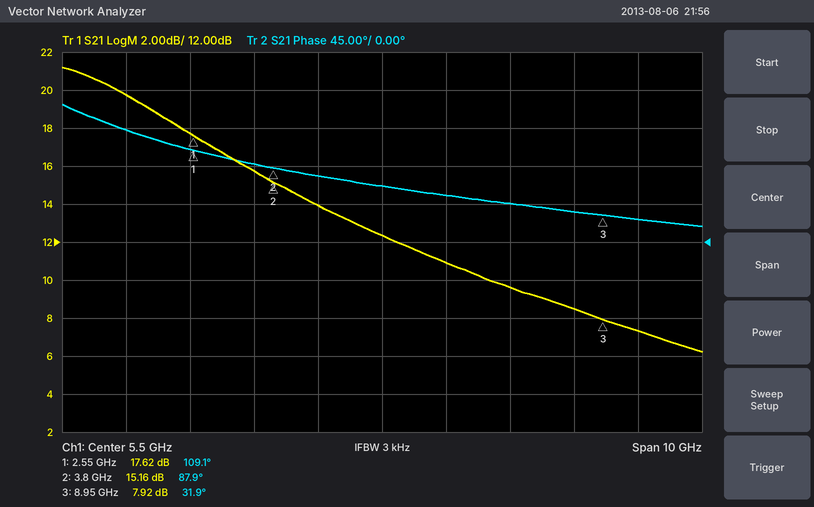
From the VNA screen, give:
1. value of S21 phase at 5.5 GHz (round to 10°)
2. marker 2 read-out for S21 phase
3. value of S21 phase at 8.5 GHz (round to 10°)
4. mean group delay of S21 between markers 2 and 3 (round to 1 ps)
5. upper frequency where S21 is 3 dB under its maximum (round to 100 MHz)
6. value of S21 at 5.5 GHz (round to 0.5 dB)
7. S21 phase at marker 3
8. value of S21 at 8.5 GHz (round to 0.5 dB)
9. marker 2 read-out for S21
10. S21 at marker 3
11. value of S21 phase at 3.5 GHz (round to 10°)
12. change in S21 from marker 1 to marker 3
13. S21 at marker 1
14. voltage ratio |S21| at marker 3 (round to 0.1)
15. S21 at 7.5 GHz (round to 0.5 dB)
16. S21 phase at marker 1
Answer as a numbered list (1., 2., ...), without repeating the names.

1. 70°
2. 87.9°
3. 40°
4. 30 ps
5. 2.3 GHz
6. 12.5 dB
7. 31.9°
8. 8.5 dB
9. 15.16 dB
10. 7.92 dB
11. 90°
12. -9.70 dB
13. 17.62 dB
14. 2.5
15. 9.5 dB
16. 109.1°
